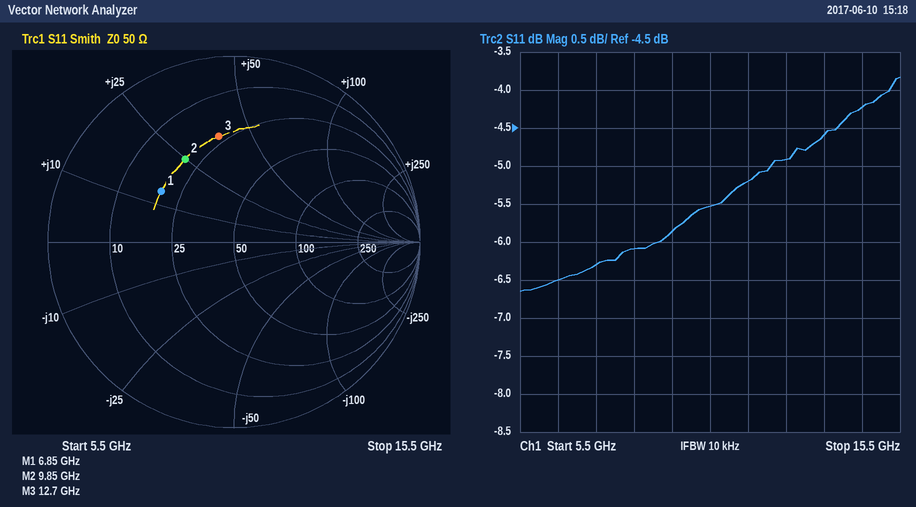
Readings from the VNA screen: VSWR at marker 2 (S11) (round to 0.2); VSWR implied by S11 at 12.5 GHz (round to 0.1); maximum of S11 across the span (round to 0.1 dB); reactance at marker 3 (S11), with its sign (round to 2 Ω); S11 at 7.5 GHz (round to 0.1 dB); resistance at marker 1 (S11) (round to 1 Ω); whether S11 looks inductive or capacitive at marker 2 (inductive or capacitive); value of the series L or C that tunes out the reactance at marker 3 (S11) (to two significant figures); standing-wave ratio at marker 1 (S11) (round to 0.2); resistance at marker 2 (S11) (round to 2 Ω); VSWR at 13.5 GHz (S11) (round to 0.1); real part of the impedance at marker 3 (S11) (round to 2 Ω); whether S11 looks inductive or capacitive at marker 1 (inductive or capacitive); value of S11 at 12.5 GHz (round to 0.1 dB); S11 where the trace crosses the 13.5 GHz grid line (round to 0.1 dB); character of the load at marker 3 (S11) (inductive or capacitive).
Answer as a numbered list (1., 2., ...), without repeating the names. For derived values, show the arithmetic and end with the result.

1. 3.2
2. |Γ| = 10^(-4.9/20) = 0.5689; VSWR = (1 + 0.5689)/(1 − 0.5689) ≈ 3.6
3. -3.8 dB
4. +38 Ω
5. -6.3 dB
6. 19 Ω
7. inductive
8. C = 1/(2π × 12.7 GHz × 38 Ω) ≈ 330 fF
9. 2.8
10. 20 Ω
11. |Γ| = 10^(-4.6/20) = 0.5888; VSWR = (1 + 0.5888)/(1 − 0.5888) ≈ 3.9
12. 22 Ω
13. inductive
14. -4.9 dB
15. -4.6 dB
16. inductive
